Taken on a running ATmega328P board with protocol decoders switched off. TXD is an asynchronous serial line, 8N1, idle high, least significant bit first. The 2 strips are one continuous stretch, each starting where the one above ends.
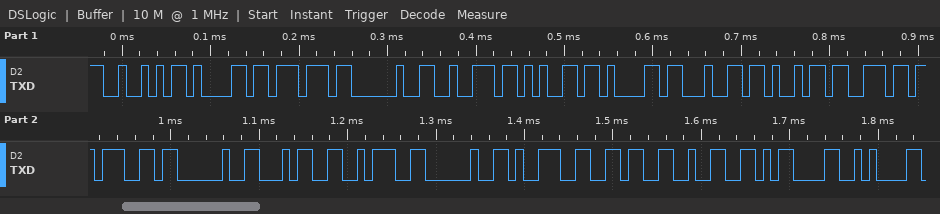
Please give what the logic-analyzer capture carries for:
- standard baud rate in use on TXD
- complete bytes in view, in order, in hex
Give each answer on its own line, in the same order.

115200 baud
0x52 0x61 0x77 0x20 0x72 0x65 0x61 0x64 0x69 0x6E 0x67 0x20 0x34 0x3A 0x20 0x39 0x36 0x32 0x0D 0x0A
